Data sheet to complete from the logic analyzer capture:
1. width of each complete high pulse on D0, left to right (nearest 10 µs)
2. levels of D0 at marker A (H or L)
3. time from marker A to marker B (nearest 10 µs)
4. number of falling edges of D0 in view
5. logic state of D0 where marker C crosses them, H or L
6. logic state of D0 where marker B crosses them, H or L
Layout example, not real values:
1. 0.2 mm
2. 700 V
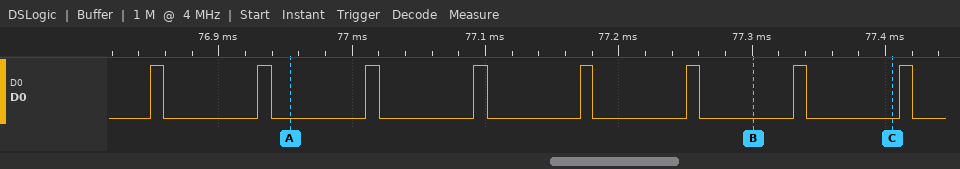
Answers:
1. 10 µs, 10 µs, 10 µs, 10 µs, 10 µs, 10 µs, 10 µs, 10 µs
2. D0=L
3. 350 µs
4. 8
5. D0=L
6. D0=L
